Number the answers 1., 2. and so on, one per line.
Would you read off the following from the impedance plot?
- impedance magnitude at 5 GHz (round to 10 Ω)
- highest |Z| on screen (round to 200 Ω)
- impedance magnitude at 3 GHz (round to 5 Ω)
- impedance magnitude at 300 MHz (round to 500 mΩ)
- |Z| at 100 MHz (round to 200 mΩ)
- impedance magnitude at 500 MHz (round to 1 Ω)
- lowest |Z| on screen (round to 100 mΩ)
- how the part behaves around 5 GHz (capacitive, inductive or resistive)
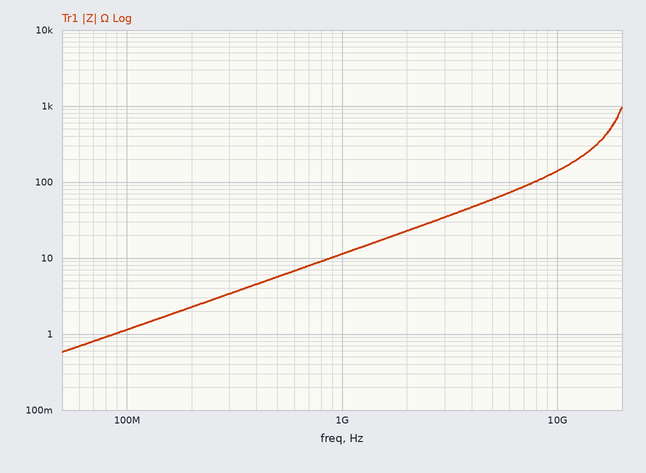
1. 60 Ω
2. 1.0 kΩ
3. 35 Ω
4. 3.5 Ω
5. 1.2 Ω
6. 6 Ω
7. 600 mΩ
8. inductive
